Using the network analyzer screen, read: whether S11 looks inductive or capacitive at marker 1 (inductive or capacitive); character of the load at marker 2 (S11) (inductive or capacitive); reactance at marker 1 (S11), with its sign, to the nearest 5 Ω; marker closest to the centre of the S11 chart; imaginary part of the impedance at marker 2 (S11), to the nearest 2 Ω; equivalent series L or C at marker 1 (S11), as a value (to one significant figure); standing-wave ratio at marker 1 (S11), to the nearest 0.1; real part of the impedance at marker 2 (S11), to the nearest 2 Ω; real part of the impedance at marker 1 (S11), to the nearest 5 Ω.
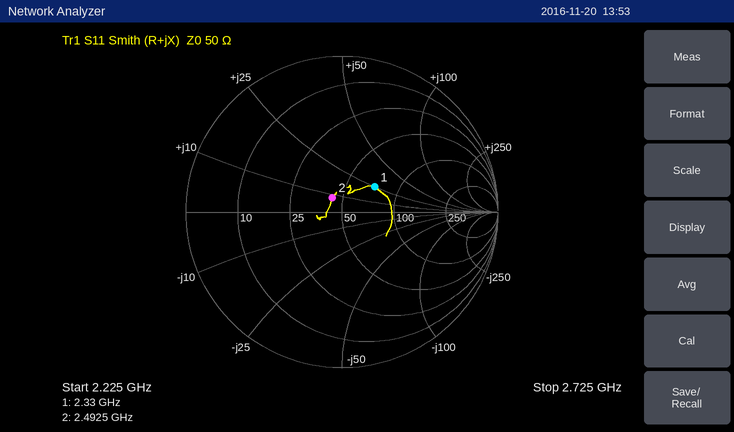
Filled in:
inductive
inductive
+25 Ω
marker 2
+8 Ω
2 nH
1.7
44 Ω
70 Ω
